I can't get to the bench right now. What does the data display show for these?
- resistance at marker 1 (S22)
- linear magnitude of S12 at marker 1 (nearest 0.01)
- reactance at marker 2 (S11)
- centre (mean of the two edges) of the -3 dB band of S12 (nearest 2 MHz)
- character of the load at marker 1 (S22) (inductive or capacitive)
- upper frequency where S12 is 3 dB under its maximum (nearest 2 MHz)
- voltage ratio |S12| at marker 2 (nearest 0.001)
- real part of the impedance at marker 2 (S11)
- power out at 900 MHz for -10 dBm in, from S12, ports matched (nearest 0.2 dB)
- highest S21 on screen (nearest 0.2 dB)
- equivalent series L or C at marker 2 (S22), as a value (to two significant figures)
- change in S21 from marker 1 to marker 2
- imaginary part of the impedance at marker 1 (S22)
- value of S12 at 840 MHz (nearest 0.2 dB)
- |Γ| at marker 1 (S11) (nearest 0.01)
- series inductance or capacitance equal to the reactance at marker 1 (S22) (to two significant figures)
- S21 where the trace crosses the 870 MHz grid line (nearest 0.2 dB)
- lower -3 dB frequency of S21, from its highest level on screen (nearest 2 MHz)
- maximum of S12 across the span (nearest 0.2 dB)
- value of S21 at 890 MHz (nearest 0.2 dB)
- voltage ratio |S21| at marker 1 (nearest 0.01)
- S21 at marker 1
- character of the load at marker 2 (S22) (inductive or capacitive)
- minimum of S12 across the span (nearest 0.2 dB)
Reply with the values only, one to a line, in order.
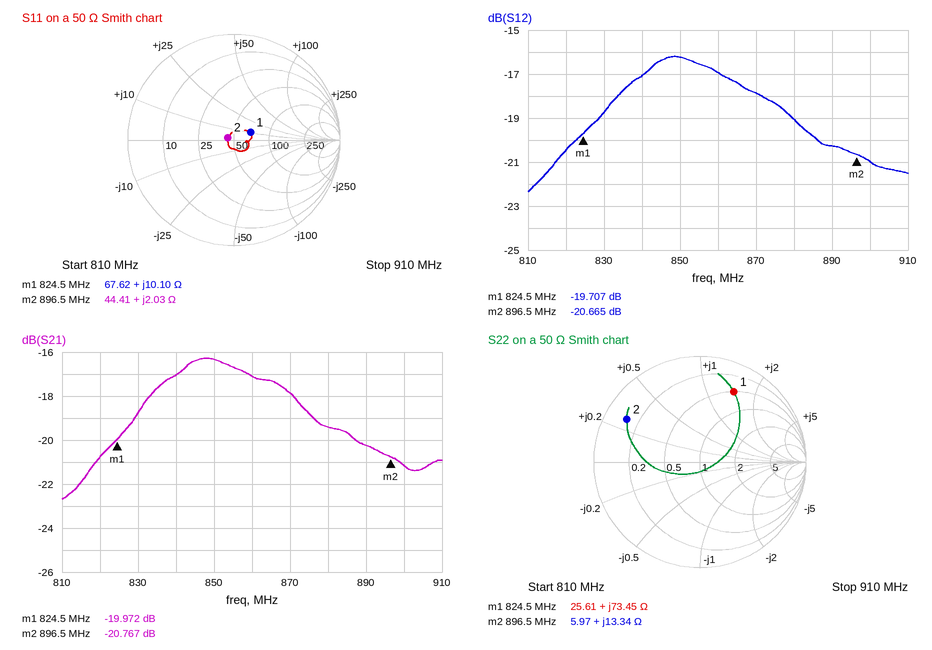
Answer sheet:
25.61 Ω
0.10
+2.03 Ω
854 MHz
inductive
880 MHz
0.093
44.41 Ω
-31.0 dBm
-16.2 dB
2.4 nH
-0.795 dB
+73.45 Ω
-17.0 dB
0.17
14 nH
-17.8 dB
828 MHz
-16.2 dB
-20.2 dB
0.10
-19.972 dB
inductive
-22.4 dB
